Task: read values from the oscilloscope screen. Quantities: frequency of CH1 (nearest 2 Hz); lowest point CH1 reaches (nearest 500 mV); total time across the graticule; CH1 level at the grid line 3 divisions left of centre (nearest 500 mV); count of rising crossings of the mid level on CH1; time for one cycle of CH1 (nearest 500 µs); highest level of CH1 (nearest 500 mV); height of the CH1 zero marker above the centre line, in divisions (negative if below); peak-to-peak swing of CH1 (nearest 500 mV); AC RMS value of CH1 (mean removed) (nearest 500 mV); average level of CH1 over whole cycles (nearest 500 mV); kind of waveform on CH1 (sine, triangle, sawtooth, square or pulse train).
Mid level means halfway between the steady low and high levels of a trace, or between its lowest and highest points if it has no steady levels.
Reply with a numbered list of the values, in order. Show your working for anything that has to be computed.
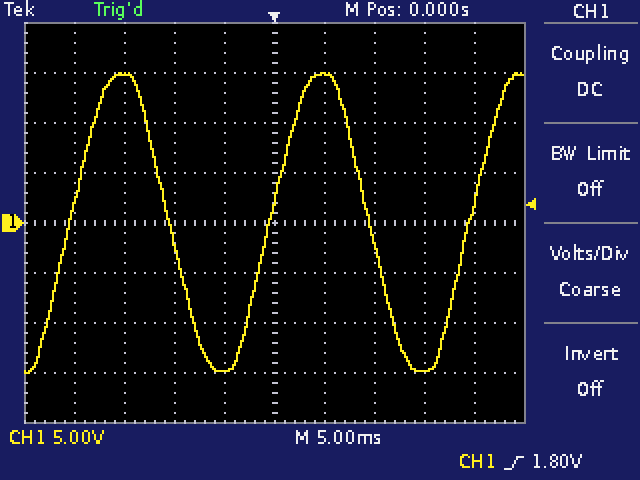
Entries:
1. 1 / 20.0 ms ≈ 50 Hz
2. -15.0 V
3. 50 ms
4. 15.0 V
5. 3
6. 20.0 ms
7. 15.0 V
8. 0.0 div
9. 15.0 V − (-15.0 V) = 30.0 V
10. 30.0 V / (2√2) ≈ 10.6 V, so 10.5 V to the nearest 500 mV
11. (15.0 V + (-15.0 V)) / 2 ≈ 0.0 V
12. sine
